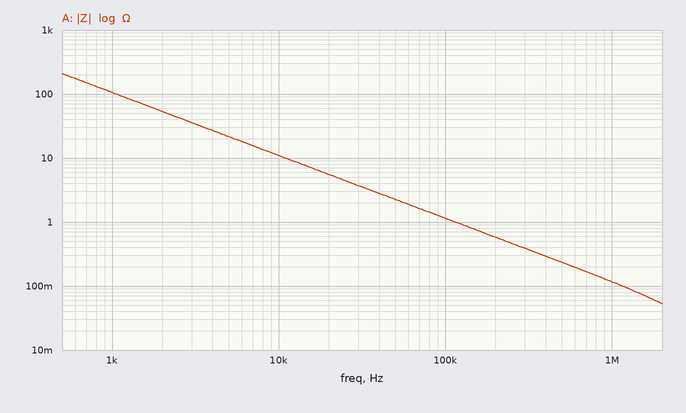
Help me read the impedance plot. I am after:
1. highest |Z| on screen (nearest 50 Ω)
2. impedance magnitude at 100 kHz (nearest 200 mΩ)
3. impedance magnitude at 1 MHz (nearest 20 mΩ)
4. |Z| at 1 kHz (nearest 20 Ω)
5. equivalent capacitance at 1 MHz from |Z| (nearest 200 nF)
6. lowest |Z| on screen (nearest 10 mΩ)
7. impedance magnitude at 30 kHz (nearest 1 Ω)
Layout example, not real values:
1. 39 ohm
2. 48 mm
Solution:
1. 200 Ω
2. 1.2 Ω
3. 120 mΩ
4. 100 Ω
5. 1.4 µF
6. 50 mΩ
7. 4 Ω
